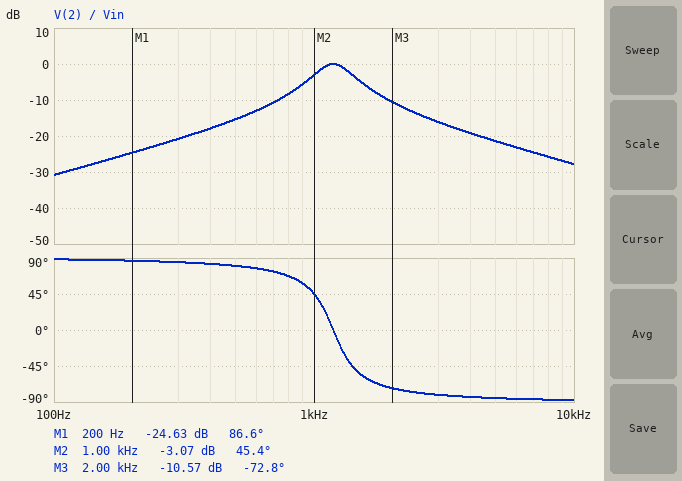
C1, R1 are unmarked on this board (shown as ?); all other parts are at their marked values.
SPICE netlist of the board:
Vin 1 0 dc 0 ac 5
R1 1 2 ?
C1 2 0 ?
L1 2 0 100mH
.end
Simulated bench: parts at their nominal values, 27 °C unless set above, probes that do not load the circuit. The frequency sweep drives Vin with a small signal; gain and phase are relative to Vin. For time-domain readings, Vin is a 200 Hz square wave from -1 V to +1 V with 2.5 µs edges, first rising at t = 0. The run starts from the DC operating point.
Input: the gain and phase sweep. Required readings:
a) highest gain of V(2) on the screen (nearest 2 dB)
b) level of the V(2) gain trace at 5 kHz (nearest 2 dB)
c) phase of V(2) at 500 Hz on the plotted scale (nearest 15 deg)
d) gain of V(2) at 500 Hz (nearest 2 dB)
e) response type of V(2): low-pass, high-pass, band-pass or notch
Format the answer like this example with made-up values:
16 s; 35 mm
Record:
0 dB; -22 dB; 75 deg; -16 dB; band-pass
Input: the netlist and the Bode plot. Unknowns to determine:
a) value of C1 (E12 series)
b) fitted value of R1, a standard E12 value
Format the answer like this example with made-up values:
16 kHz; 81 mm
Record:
180 nF; 2.2 kΩ
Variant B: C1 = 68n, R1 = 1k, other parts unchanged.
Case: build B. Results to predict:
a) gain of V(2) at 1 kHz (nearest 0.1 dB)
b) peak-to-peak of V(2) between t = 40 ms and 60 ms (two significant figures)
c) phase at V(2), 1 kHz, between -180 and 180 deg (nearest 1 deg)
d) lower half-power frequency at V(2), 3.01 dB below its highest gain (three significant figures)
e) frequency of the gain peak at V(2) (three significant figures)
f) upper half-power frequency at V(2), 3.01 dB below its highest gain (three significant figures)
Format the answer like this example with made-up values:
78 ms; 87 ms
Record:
-3.7 dB; 2.4 V; 49 deg; 1.09 kHz; 1.93 kHz; 3.43 kHz
